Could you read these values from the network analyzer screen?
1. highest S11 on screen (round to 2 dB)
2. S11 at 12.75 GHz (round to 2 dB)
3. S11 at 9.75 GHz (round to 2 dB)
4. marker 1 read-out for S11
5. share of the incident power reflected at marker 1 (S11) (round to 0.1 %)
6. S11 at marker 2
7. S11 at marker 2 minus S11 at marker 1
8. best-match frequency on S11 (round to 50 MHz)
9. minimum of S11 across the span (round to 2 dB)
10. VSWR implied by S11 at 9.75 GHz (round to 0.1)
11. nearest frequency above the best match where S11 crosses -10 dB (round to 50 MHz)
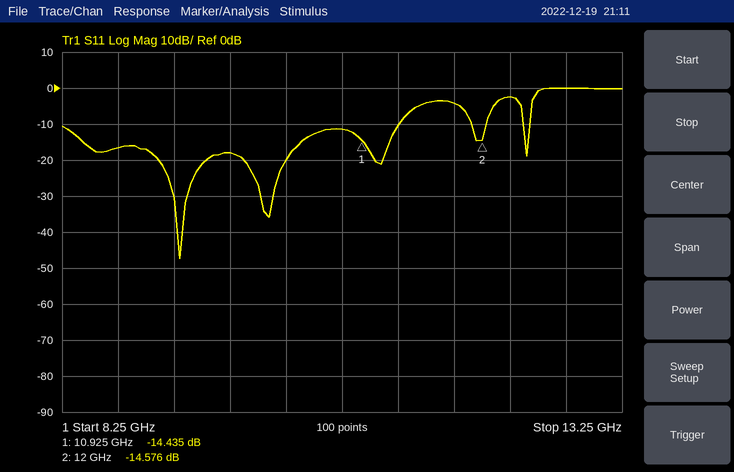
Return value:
0 dB
0 dB
-18 dB
-14.435 dB
3.6 %
-14.576 dB
-0.141 dB
9.30 GHz
-48 dB
1.3
11.25 GHz
